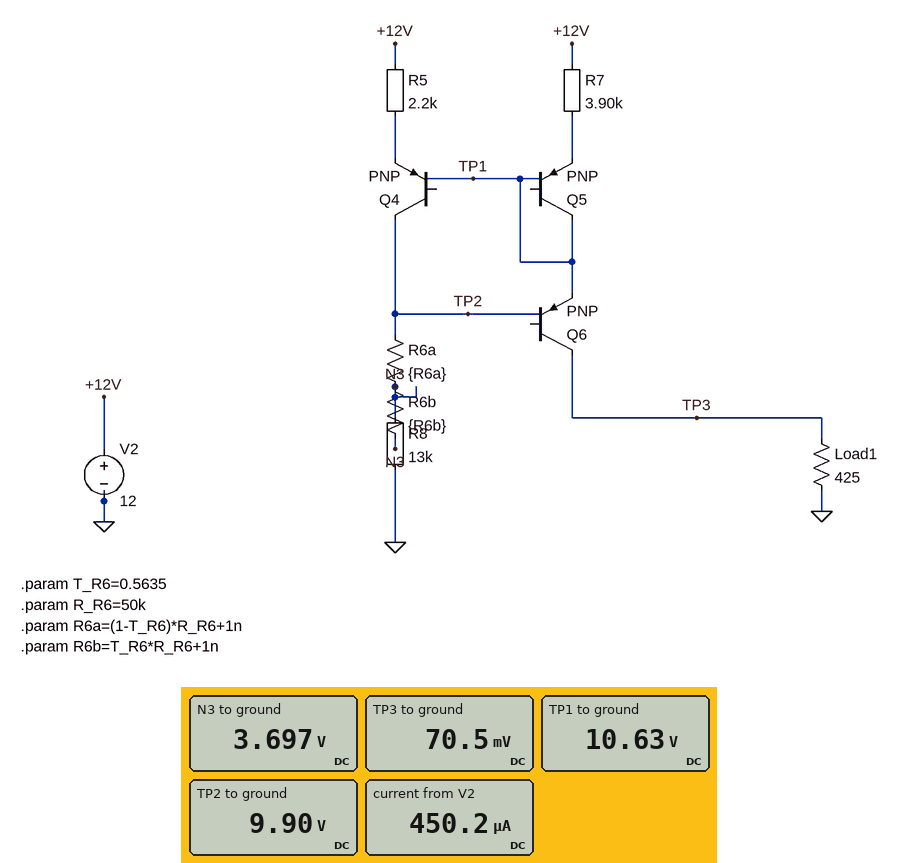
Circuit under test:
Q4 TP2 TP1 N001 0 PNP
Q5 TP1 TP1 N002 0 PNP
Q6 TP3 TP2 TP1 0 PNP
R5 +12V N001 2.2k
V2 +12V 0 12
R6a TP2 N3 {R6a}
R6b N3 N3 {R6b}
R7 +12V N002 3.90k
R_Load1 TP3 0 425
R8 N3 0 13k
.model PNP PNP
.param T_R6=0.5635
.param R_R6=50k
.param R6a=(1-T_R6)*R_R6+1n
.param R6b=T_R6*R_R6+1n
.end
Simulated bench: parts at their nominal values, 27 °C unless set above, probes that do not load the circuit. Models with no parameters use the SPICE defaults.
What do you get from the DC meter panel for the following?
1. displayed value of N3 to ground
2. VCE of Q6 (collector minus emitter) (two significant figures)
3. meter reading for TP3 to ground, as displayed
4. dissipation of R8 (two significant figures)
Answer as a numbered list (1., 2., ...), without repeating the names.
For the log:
1. 3.697 V
2. -11 V
3. 70.5 mV
4. 1.1 mW
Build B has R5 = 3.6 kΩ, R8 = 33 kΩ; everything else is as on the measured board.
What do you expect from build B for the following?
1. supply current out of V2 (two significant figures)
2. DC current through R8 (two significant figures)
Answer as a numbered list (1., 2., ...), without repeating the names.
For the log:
1. 350 µA
2. 180 µA
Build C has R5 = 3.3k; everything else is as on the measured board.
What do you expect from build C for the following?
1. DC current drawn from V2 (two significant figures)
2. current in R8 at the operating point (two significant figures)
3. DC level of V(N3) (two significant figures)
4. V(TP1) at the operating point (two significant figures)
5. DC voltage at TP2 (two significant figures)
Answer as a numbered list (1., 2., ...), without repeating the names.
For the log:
1. 510 µA
2. 280 µA
3. 3.6 V
4. 10 V
5. 9.6 V
